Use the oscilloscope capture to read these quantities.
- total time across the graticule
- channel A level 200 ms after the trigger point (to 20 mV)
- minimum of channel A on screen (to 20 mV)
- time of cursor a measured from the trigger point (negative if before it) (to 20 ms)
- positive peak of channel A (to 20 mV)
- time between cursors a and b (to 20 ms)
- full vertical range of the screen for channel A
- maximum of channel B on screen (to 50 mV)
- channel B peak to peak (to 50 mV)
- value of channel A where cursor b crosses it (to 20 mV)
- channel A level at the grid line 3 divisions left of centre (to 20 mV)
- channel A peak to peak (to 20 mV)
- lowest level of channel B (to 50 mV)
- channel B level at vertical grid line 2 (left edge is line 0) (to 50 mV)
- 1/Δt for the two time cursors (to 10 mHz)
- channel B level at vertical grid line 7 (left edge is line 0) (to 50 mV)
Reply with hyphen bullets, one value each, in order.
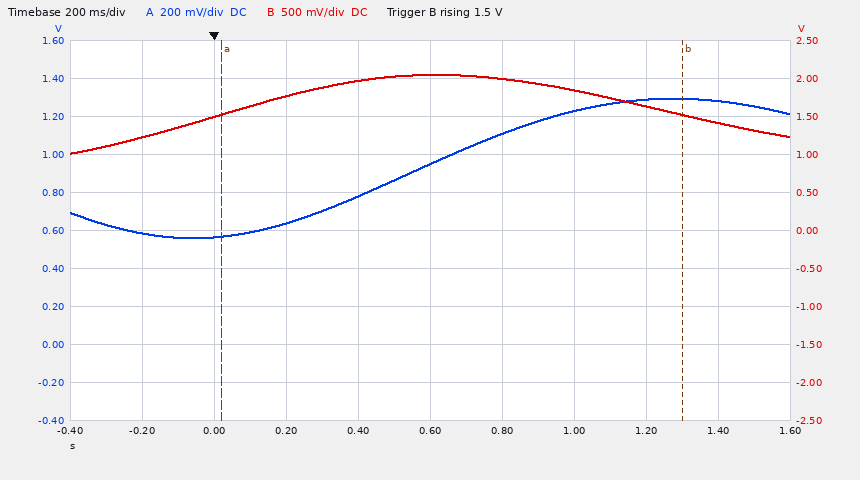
- 2 s
- 640 mV
- 560 mV
- +20 ms
- 1.30 V
- 1.28 s
- 2 V
- 2.05 V
- 1.05 V
- 1.30 V
- 560 mV
- 740 mV
- 1.00 V
- 1.50 V
- 780 mHz
- 1.85 V
